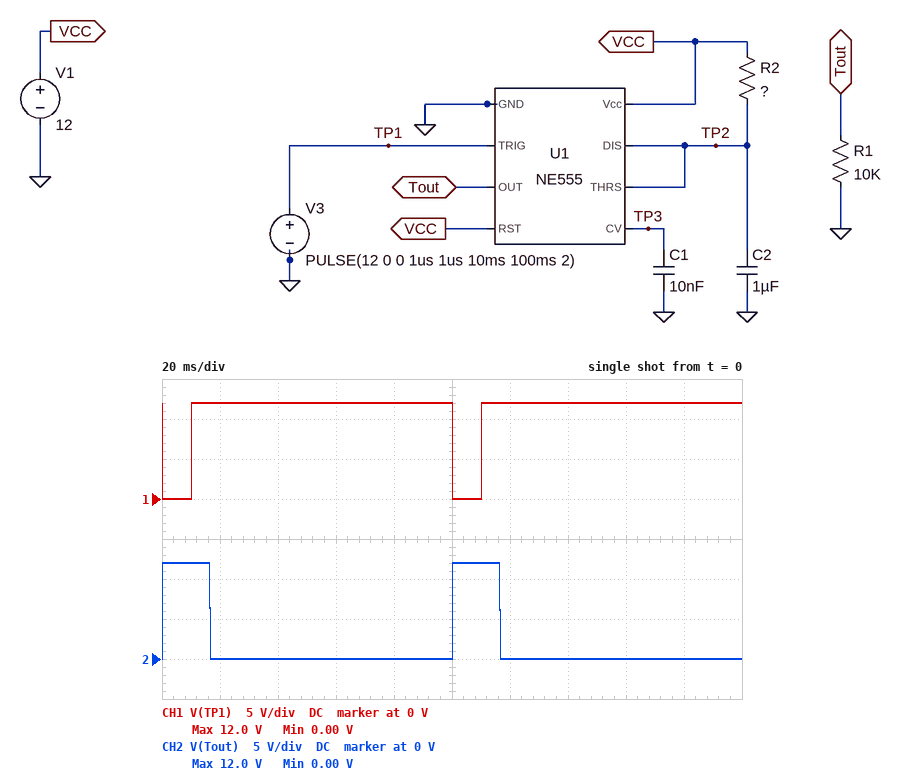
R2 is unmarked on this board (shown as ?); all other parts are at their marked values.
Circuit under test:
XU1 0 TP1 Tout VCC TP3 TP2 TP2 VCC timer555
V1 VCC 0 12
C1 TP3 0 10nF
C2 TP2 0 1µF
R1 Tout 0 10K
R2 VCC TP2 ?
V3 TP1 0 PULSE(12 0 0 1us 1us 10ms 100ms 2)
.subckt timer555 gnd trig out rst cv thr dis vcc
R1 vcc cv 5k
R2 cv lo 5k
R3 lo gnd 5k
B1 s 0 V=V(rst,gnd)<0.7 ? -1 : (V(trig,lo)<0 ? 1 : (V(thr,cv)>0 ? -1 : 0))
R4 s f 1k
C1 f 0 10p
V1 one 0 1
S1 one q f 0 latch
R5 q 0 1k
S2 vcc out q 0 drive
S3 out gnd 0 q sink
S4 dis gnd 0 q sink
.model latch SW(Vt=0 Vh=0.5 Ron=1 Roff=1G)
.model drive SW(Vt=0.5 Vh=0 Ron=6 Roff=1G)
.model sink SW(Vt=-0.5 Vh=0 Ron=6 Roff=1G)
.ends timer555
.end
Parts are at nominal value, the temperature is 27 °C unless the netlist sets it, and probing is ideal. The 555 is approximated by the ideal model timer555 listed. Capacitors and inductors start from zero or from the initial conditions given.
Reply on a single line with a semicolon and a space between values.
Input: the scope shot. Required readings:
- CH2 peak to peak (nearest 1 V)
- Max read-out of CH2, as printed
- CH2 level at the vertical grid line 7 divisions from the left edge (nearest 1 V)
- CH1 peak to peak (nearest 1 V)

12 V; 12.0 V; 0 V; 12 V
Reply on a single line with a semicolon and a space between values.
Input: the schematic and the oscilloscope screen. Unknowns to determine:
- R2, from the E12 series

15 kΩ
